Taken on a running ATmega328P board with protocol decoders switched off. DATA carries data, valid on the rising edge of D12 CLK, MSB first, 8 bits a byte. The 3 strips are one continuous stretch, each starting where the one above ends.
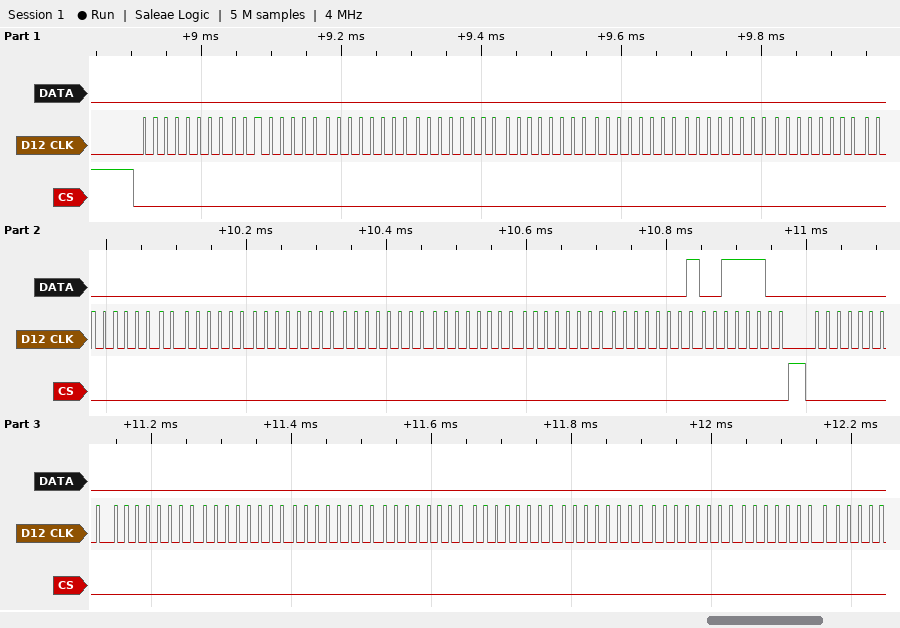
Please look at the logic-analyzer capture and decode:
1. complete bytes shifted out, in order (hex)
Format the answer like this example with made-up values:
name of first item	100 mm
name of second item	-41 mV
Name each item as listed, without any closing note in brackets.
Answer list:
complete bytes shifted out, in order	00 00 00 00 00 00 00 00 00 00 00 00 00 00 01 3C 00 00 00 00 00 00 00 00 00
